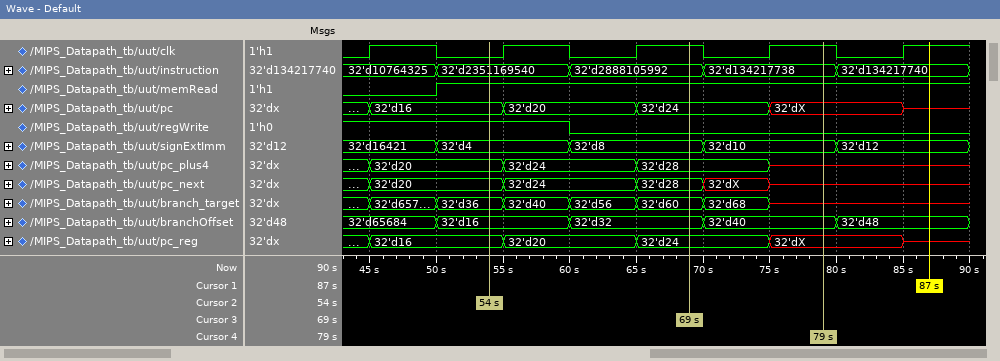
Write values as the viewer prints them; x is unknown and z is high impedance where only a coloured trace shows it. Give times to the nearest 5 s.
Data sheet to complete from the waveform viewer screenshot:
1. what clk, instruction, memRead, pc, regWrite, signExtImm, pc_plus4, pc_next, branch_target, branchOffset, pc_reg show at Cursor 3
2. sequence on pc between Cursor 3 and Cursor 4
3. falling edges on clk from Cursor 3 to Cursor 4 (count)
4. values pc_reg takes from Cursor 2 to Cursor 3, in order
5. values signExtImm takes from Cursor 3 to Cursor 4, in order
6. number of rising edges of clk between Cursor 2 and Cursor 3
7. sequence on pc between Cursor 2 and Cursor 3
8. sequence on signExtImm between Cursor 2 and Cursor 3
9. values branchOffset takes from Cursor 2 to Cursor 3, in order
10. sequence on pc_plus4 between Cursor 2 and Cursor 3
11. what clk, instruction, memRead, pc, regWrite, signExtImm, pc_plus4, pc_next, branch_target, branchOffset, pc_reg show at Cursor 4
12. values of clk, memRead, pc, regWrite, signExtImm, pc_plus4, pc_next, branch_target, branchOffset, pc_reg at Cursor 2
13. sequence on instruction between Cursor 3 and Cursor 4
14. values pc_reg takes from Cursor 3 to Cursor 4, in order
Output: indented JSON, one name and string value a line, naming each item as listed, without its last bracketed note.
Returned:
{
  "what clk, instruction, memRead, pc, regWrite, signExtImm, pc_plus4, pc_next, branch_target, branchOffset, pc_reg show at Cursor 3": "clk=1, instruction=32'd2888105992, memRead=1, pc=32'd24, regWrite=0, signExtImm=32'd8, pc_plus4=32'd28, pc_next=32'd28, branch_target=32'd60, branchOffset=32'd32, pc_reg=32'd24",
  "sequence on pc between Cursor 3 and Cursor 4": "32'd24, 32'dX",
  "falling edges on clk from Cursor 3 to Cursor 4": "1",
  "values pc_reg takes from Cursor 2 to Cursor 3, in order": "32'd16, 32'd20, 32'd24",
  "values signExtImm takes from Cursor 3 to Cursor 4, in order": "32'd8, 32'd10",
  "number of rising edges of clk between Cursor 2 and Cursor 3": "2",
  "sequence on pc between Cursor 2 and Cursor 3": "32'd16, 32'd20, 32'd24",
  "sequence on signExtImm between Cursor 2 and Cursor 3": "32'd4, 32'd8",
  "values branchOffset takes from Cursor 2 to Cursor 3, in order": "32'd16, 32'd32",
  "sequence on pc_plus4 between Cursor 2 and Cursor 3": "32'd20, 32'd24, 32'd28",
  "what clk, instruction, memRead, pc, regWrite, signExtImm, pc_plus4, pc_next, branch_target, branchOffset, pc_reg show at Cursor 4": "clk=1, instruction=32'd134217738, memRead=1, pc=32'dX, regWrite=0, signExtImm=32'd10, pc_plus4=x, pc_next=x, branch_target=x, branchOffset=32'd40, pc_reg=32'dX",
  "values of clk, memRead, pc, regWrite, signExtImm, pc_plus4, pc_next, branch_target, branchOffset, pc_reg at Cursor 2": "clk=0, memRead=1, pc=32'd16, regWrite=1, signExtImm=32'd4, pc_plus4=32'd20, pc_next=32'd20, branch_target=32'd36, branchOffset=32'd16, pc_reg=32'd16",
  "sequence on instruction between Cursor 3 and Cursor 4": "32'd2888105992, 32'd134217738",
  "values pc_reg takes from Cursor 3 to Cursor 4, in order": "32'd24, 32'dX"
}
